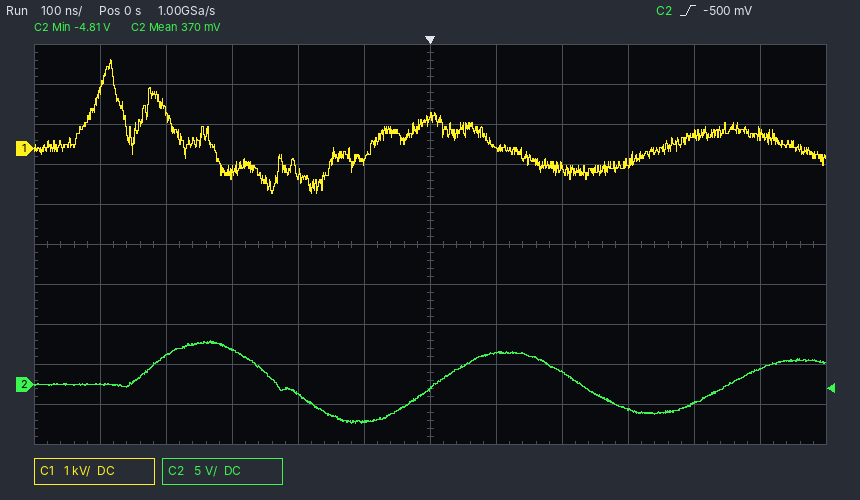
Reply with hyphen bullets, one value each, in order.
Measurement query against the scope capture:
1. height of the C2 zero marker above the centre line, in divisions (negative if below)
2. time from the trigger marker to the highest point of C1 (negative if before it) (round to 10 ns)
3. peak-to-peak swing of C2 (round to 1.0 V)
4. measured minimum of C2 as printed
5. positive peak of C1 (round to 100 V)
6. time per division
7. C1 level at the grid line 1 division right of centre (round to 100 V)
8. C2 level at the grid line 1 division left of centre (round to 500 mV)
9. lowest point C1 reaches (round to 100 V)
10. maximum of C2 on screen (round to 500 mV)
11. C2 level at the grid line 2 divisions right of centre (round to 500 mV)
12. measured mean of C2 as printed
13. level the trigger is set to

- -3.5 div
- -480 ns
- 10.0 V
- -4.81 V
- 2.2 kV
- 100 ns
- 0.0 kV
- -4.5 V
- -1.1 kV
- 5.5 V
- 1.5 V
- 370 mV
- -500 mV
